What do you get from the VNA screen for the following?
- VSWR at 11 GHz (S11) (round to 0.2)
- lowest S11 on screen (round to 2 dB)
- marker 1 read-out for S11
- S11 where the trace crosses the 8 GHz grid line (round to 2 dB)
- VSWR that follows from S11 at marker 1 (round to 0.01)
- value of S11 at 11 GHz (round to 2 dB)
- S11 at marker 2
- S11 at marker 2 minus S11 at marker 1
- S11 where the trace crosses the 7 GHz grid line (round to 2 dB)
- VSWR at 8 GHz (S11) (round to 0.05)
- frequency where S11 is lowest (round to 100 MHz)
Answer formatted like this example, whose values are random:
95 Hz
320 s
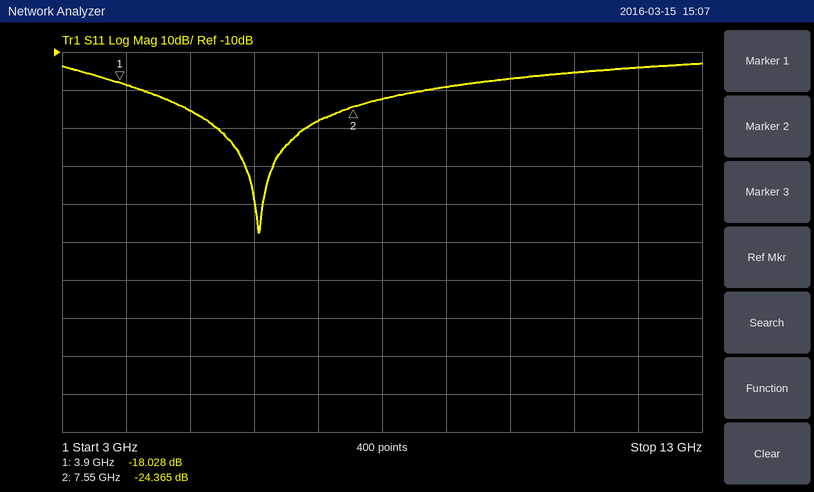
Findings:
1.4
-58 dB
-18.028 dB
-22 dB
1.29
-16 dB
-24.365 dB
-6.337 dB
-28 dB
1.15
6.1 GHz
